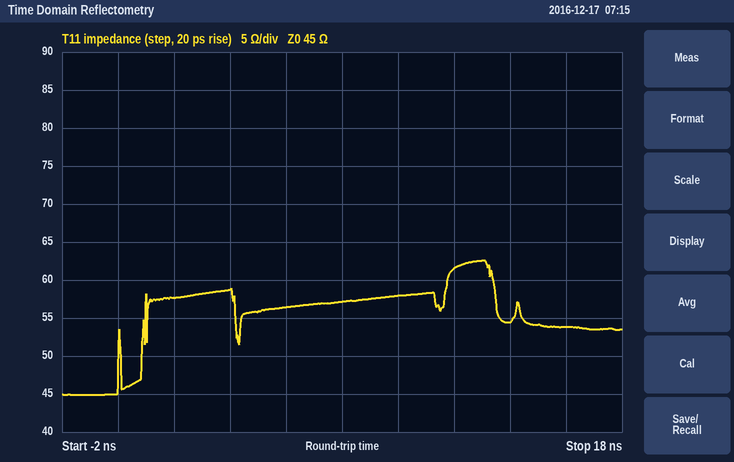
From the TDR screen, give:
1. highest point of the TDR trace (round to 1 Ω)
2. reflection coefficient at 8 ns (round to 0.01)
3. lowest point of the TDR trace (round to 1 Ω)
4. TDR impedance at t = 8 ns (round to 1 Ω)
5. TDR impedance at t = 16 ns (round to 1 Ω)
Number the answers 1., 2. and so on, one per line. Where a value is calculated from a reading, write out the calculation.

1. 63 Ω
2. (57 − 45)/(57 + 45) ≈ +0.12
3. 45 Ω
4. 57 Ω
5. 54 Ω
